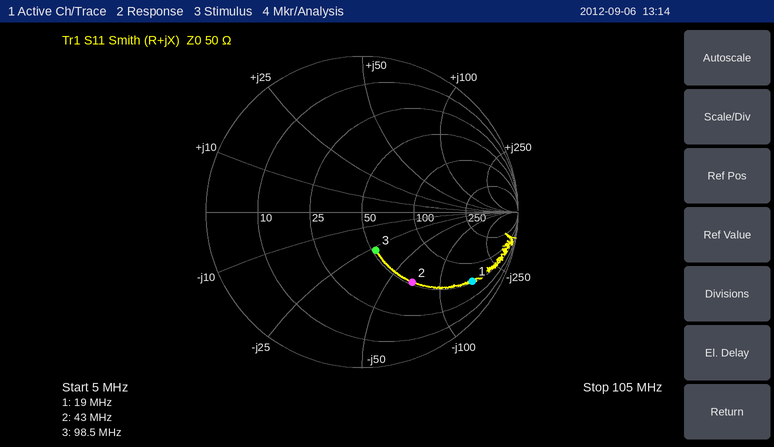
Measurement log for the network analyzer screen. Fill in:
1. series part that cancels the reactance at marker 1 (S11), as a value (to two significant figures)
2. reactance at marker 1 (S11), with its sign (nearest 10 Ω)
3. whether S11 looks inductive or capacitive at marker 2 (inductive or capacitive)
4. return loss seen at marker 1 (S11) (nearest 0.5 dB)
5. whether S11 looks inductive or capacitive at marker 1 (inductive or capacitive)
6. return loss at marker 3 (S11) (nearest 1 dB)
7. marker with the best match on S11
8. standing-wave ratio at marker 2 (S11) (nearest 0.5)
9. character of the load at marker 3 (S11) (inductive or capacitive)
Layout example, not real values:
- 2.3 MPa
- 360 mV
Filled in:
- 1.3 µH
- -160 Ω
- capacitive
- 1.5 dB
- capacitive
- 12 dB
- marker 3
- 3.5
- capacitive
